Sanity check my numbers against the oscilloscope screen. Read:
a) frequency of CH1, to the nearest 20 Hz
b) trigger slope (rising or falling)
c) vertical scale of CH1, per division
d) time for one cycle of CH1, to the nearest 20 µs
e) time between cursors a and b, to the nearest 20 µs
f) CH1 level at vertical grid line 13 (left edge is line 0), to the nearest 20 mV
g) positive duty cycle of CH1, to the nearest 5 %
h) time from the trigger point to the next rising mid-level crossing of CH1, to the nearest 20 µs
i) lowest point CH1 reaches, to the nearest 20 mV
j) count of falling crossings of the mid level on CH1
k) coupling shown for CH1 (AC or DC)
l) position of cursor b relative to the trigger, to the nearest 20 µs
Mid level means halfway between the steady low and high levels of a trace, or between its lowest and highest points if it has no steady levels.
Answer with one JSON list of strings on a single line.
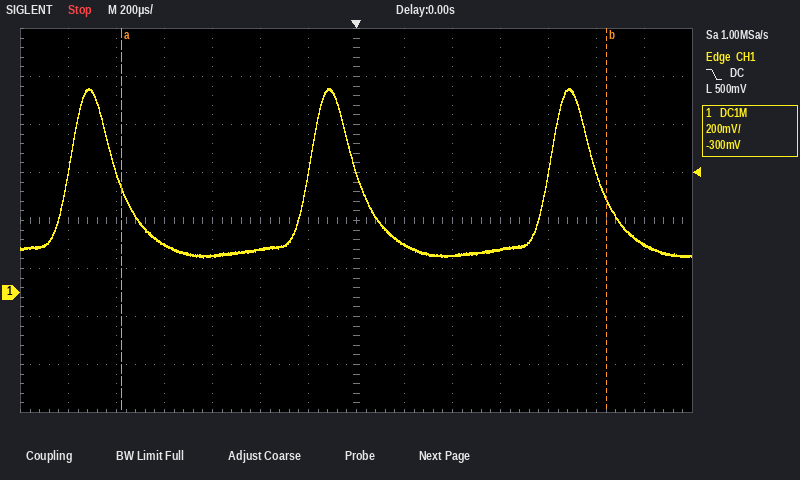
["1.00 kHz", "falling", "200 mV", "1.00 ms", "2.02 ms", "200 mV", "20 %", "800 µs", "140 mV", "3", "DC", "+1.04 ms"]
